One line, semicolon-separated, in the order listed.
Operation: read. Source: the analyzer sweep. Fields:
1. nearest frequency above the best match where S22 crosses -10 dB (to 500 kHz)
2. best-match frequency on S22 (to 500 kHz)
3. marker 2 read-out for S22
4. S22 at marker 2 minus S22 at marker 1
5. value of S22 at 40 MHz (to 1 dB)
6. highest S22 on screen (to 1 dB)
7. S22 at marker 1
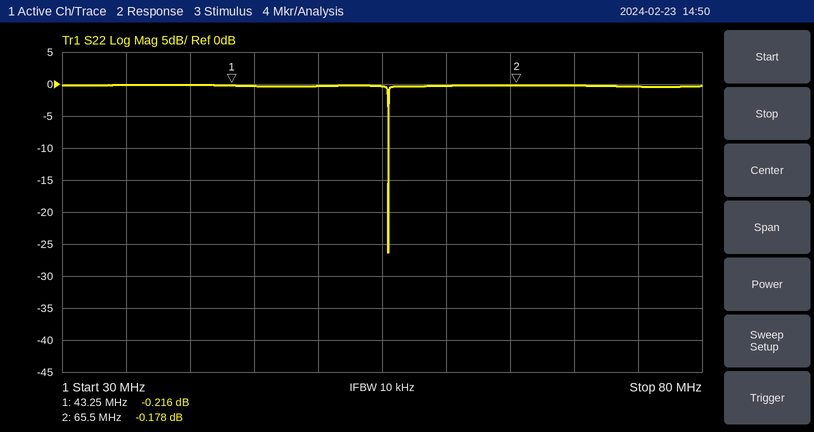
55.5 MHz; 55.5 MHz; -0.178 dB; 0.038 dB; 0 dB; 0 dB; -0.216 dB
